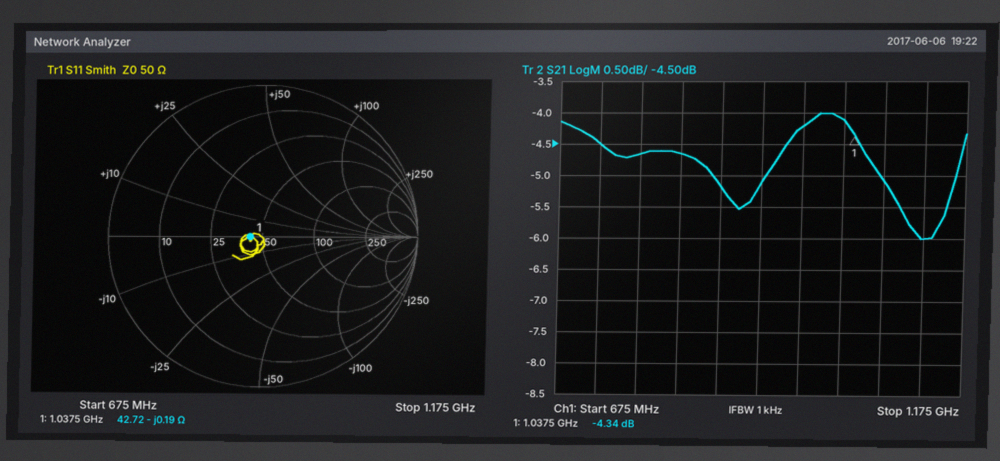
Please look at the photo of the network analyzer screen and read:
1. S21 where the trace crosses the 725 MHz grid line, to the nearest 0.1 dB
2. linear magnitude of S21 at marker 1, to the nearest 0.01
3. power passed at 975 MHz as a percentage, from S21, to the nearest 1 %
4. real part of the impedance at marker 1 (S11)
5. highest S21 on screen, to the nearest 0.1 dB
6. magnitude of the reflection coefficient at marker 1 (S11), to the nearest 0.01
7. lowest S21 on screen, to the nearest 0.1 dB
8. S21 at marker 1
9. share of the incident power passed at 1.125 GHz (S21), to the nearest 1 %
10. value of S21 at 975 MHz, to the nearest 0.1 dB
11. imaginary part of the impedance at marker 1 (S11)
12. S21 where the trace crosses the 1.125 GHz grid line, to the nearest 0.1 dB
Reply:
-4.5 dB
0.61
38 %
42.72 Ω
-4.0 dB
0.08
-6.0 dB
-4.34 dB
25 %
-4.2 dB
-0.19 Ω
-6.0 dB
